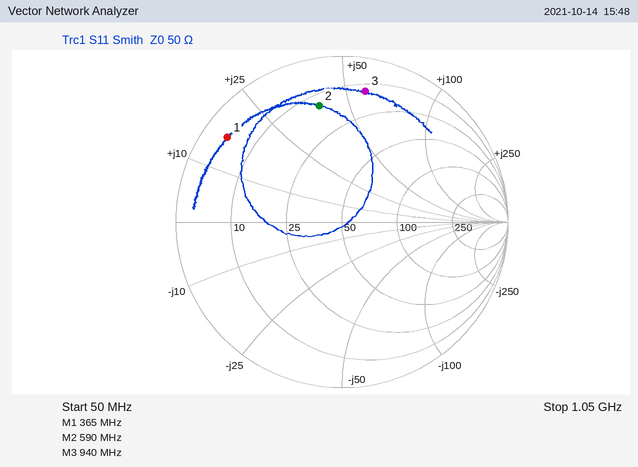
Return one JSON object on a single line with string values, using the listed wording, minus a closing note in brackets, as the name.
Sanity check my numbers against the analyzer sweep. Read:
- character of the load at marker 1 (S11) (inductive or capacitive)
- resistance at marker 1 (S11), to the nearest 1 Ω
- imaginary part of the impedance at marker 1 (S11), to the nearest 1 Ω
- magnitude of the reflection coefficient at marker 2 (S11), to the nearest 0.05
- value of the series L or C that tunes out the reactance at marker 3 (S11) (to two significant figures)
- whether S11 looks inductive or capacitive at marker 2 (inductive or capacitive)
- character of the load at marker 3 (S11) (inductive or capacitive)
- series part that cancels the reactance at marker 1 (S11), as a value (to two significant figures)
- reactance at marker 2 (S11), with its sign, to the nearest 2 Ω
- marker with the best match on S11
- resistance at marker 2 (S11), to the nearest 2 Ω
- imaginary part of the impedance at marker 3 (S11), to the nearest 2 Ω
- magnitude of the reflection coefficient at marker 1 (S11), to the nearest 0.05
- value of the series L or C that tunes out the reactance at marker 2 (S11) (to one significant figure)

{"character of the load at marker 1 (S11)": "inductive", "resistance at marker 1 (S11), to the nearest 1 Ω": "4 Ω", "imaginary part of the impedance at marker 1 (S11), to the nearest 1 Ω": "+16 Ω", "magnitude of the reflection coefficient at marker 2 (S11), to the nearest 0.05": "0.70", "value of the series L or C that tunes out the reactance at marker 3 (S11)": "2.9 pF", "whether S11 looks inductive or capacitive at marker 2": "inductive", "character of the load at marker 3 (S11)": "inductive", "series part that cancels the reactance at marker 1 (S11), as a value": "27 pF", "reactance at marker 2 (S11), with its sign, to the nearest 2 Ω": "+40 Ω", "marker with the best match on S11": "marker 2", "resistance at marker 2 (S11), to the nearest 2 Ω": "14 Ω", "imaginary part of the impedance at marker 3 (S11), to the nearest 2 Ω": "+58 Ω", "magnitude of the reflection coefficient at marker 1 (S11), to the nearest 0.05": "0.85", "value of the series L or C that tunes out the reactance at marker 2 (S11)": "7 pF"}
